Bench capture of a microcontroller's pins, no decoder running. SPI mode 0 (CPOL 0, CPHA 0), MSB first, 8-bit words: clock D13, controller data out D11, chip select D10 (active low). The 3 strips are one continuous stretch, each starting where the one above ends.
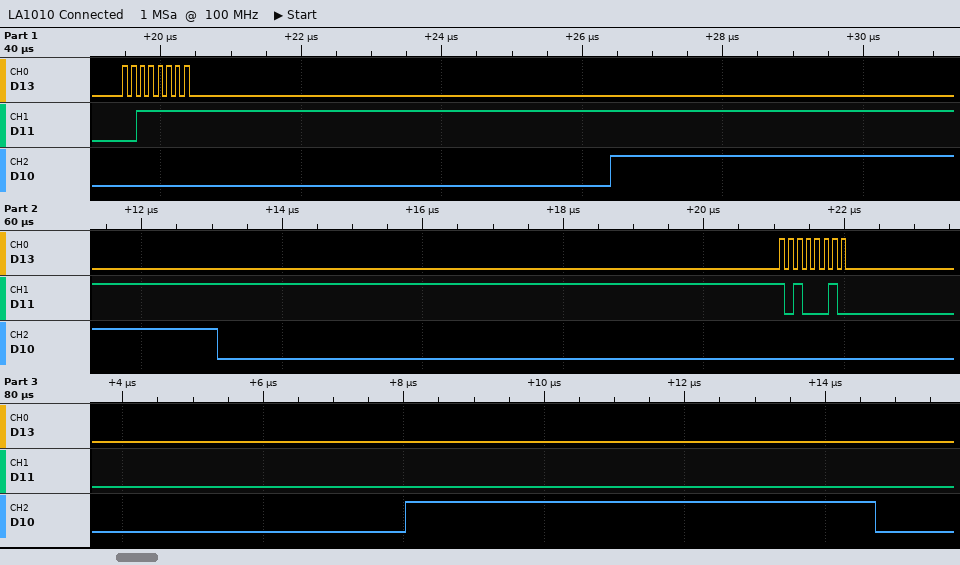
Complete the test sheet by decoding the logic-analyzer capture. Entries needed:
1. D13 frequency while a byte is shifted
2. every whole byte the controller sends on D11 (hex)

8 MHz
3F A2
